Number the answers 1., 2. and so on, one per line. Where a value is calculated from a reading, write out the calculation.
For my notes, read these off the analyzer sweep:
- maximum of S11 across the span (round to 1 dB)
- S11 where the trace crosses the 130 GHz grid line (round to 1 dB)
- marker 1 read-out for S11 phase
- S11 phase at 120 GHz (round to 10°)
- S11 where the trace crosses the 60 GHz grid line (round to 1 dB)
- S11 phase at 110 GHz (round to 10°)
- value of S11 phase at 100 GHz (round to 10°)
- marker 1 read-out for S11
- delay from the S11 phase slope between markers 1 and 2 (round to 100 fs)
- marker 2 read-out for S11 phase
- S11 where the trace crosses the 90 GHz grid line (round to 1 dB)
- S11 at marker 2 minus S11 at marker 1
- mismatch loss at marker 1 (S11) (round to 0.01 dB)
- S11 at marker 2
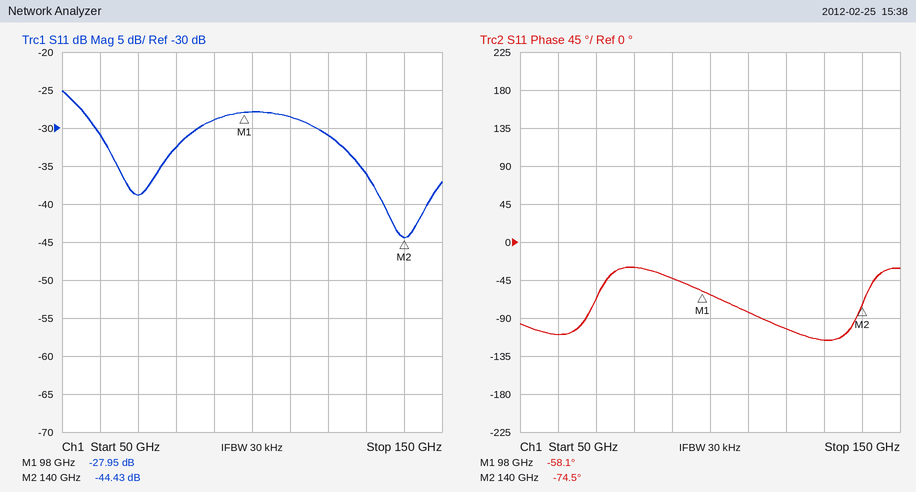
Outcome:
1. -25 dB
2. -36 dB
3. -58.1°
4. -100°
5. -31 dB
6. -80°
7. -60°
8. -27.95 dB
9. −(-74.5° − (-58.1°))/(360° × 42 GHz) ≈ 1.1 ps
10. -74.5°
11. -29 dB
12. -44.43 − (-27.95) = -16.48 dB
13. −10 log10(1 − 10^(-27.95/10)) ≈ 0.01 dB
14. -44.43 dB
